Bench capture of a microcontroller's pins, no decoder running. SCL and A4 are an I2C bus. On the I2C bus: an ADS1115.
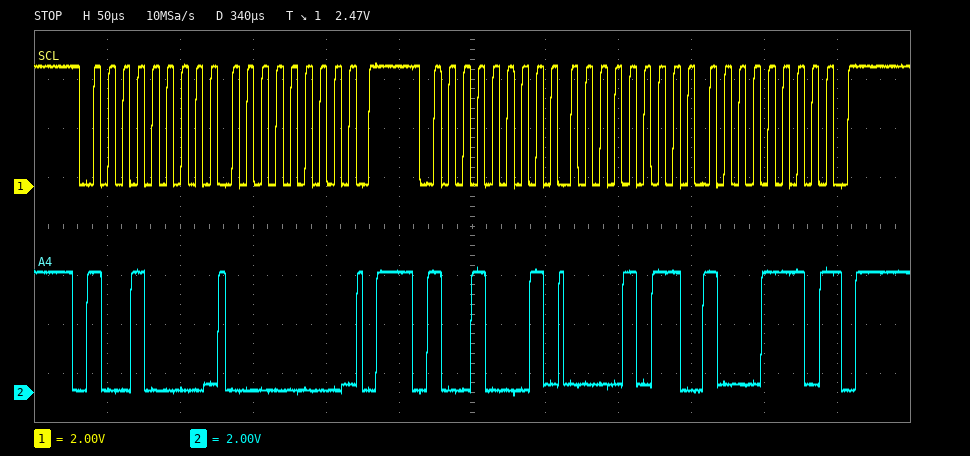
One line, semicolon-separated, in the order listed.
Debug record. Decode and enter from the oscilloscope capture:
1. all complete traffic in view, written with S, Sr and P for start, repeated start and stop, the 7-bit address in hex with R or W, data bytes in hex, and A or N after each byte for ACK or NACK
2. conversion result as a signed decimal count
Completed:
S 48W A 00 A P S 48R A 0B A 8E N P; 2958
